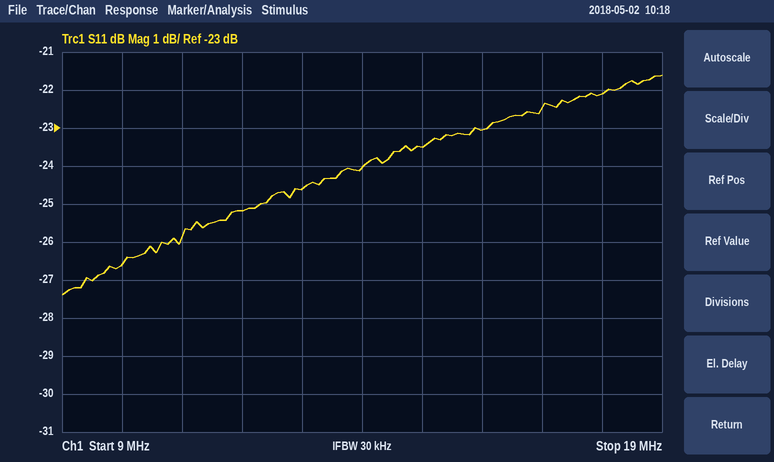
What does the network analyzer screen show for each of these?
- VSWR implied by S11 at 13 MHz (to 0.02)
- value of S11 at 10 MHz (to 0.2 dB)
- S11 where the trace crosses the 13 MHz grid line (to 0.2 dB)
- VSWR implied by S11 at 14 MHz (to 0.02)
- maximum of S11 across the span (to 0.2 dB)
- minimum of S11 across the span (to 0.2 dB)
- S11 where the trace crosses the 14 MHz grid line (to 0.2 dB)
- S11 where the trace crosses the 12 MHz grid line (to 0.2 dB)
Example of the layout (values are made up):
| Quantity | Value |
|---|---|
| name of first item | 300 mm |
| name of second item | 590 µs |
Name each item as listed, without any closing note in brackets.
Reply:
| Quantity | Value |
|---|---|
| VSWR implied by S11 at 13 MHz | 1.12 |
| value of S11 at 10 MHz | -26.6 dB |
| S11 where the trace crosses the 13 MHz grid line | -24.6 dB |
| VSWR implied by S11 at 14 MHz | 1.14 |
| maximum of S11 across the span | -21.6 dB |
| minimum of S11 across the span | -27.4 dB |
| S11 where the trace crosses the 14 MHz grid line | -24.0 dB |
| S11 where the trace crosses the 12 MHz grid line | -25.2 dB |
